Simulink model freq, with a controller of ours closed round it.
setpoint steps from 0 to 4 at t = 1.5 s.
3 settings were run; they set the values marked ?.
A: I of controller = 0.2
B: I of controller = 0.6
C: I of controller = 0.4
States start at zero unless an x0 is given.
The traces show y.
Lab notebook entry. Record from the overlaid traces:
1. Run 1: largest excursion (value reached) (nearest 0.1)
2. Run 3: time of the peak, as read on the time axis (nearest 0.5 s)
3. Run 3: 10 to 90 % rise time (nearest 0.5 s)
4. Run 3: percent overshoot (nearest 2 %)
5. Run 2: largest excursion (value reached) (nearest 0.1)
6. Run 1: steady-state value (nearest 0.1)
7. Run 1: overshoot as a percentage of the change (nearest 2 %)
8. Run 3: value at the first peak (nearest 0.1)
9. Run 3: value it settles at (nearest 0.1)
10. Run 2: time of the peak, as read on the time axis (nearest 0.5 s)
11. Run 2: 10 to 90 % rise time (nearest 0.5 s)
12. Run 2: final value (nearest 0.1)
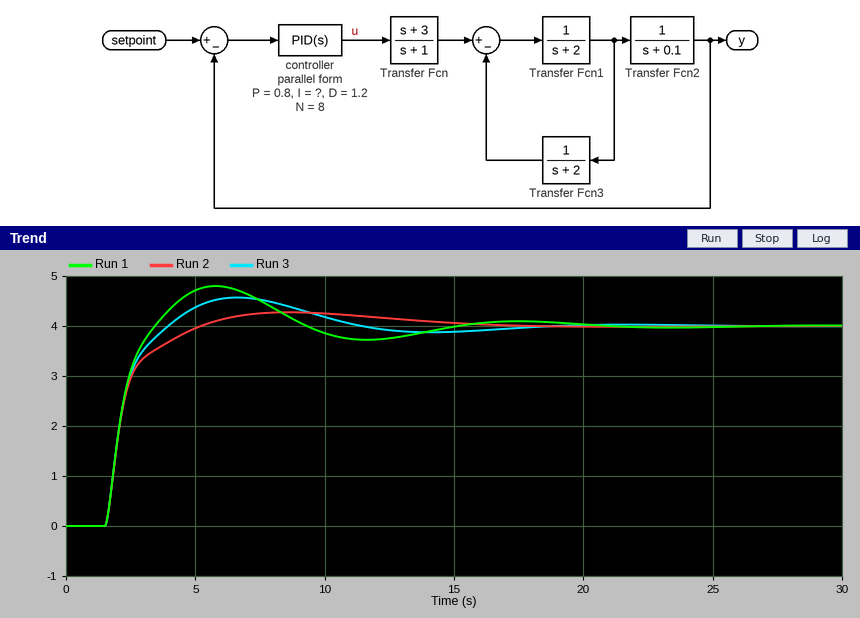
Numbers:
4.8
6.5 s
1.5 s
14 %
4.3
4.0
20 %
4.6
4.0
8.5 s
2.0 s
4.0
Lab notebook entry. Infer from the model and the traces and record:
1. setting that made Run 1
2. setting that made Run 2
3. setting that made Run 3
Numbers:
B
A
C
